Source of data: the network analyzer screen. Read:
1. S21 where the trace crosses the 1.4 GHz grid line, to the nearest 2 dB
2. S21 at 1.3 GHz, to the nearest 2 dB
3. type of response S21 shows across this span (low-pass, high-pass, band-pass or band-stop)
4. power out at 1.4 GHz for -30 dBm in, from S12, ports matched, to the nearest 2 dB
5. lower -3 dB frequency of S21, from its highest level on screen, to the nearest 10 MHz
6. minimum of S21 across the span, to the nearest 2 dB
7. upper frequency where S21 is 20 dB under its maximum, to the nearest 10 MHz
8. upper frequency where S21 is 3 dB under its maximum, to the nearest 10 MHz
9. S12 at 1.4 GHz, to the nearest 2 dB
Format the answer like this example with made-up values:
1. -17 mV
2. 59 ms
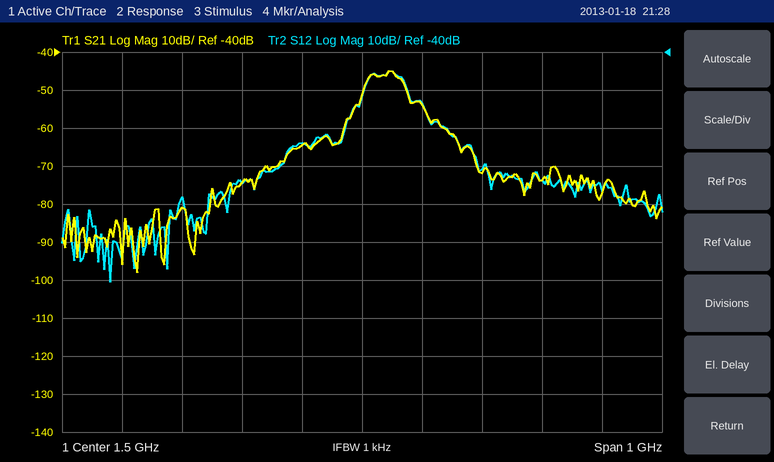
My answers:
1. -64 dB
2. -74 dB
3. band-pass
4. -94 dBm
5. 1.51 GHz
6. -98 dB
7. 1.66 GHz
8. 1.57 GHz
9. -64 dB
